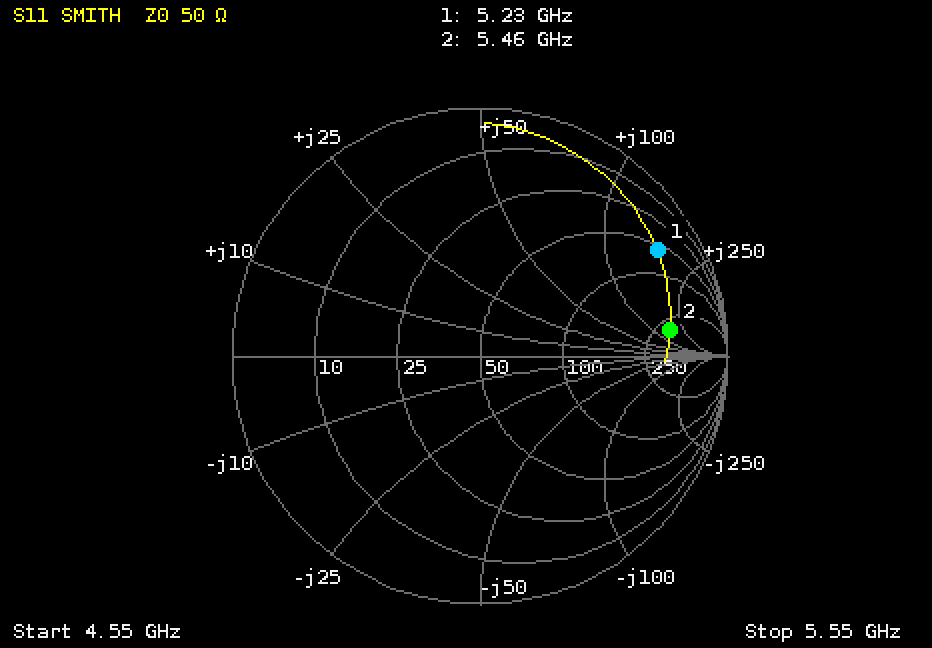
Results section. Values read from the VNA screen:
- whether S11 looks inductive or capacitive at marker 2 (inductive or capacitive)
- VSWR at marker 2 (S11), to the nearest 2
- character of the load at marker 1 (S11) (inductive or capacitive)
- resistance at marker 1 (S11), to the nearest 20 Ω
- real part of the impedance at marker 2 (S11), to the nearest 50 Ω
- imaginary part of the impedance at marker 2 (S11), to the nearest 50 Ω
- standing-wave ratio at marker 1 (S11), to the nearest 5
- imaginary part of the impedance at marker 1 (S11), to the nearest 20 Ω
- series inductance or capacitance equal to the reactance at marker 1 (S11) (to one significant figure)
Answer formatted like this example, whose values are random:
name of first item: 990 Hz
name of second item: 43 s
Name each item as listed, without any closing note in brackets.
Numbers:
whether S11 looks inductive or capacitive at marker 2: inductive
VSWR at marker 2 (S11), to the nearest 2: 8
character of the load at marker 1 (S11): inductive
resistance at marker 1 (S11), to the nearest 20 Ω: 60 Ω
real part of the impedance at marker 2 (S11), to the nearest 50 Ω: 300 Ω
imaginary part of the impedance at marker 2 (S11), to the nearest 50 Ω: +150 Ω
standing-wave ratio at marker 1 (S11), to the nearest 5: 10
imaginary part of the impedance at marker 1 (S11), to the nearest 20 Ω: +160 Ω
series inductance or capacitance equal to the reactance at marker 1 (S11): 5 nH
